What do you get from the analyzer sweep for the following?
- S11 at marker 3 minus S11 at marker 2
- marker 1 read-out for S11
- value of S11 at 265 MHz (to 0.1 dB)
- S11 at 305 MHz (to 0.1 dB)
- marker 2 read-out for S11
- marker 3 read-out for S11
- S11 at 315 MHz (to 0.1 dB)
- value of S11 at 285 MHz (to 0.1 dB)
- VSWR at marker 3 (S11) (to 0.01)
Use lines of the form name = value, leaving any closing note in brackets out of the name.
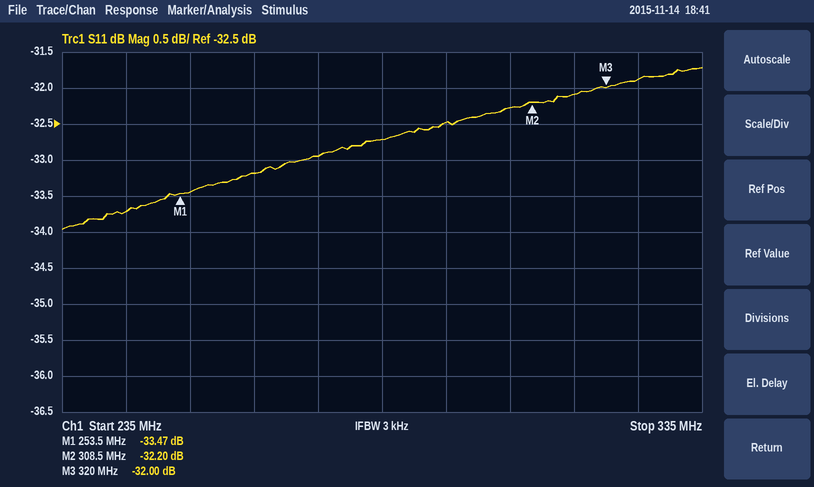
S11 at marker 3 minus S11 at marker 2 = 0.20 dB
marker 1 read-out for S11 = -33.47 dB
value of S11 at 265 MHz = -33.2 dB
S11 at 305 MHz = -32.3 dB
marker 2 read-out for S11 = -32.20 dB
marker 3 read-out for S11 = -32.00 dB
S11 at 315 MHz = -32.1 dB
value of S11 at 285 MHz = -32.7 dB
VSWR at marker 3 (S11) = 1.05
